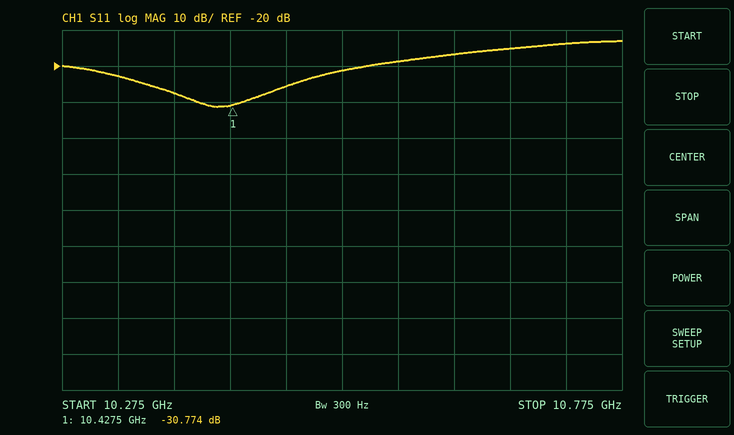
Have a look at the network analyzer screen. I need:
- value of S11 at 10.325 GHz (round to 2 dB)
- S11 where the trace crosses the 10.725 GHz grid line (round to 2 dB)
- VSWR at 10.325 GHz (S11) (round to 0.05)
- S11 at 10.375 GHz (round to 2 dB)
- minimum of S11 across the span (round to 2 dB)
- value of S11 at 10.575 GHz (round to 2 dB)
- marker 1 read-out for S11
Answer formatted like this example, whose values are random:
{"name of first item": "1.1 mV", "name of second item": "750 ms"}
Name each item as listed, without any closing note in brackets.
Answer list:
{"value of S11 at 10.325 GHz": "-22 dB", "S11 where the trace crosses the 10.725 GHz grid line": "-14 dB", "VSWR at 10.325 GHz (S11)": "1.15", "S11 at 10.375 GHz": "-28 dB", "minimum of S11 across the span": "-32 dB", "value of S11 at 10.575 GHz": "-18 dB", "marker 1 read-out for S11": "-30.774 dB"}
